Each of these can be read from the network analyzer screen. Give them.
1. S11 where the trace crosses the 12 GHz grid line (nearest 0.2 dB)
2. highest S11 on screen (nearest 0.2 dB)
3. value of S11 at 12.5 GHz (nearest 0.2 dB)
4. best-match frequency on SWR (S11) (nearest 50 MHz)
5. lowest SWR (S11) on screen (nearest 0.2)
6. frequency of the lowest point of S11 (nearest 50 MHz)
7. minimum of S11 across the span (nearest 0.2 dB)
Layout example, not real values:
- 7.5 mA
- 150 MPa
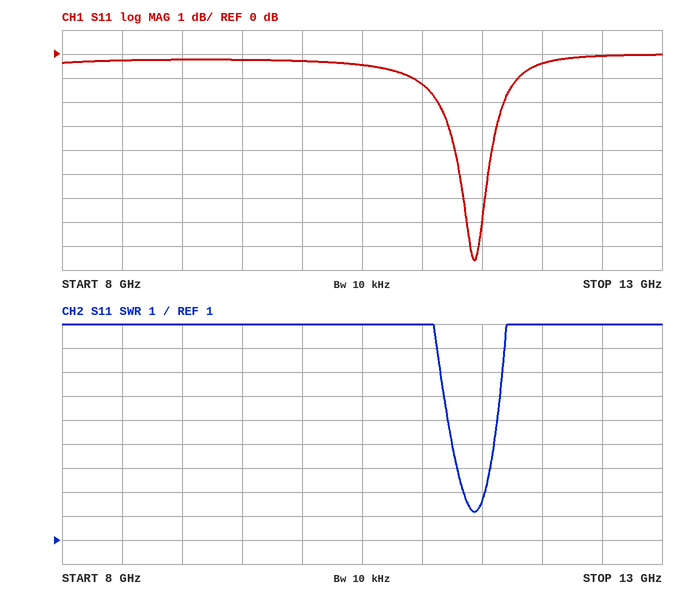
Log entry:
- -0.4 dB
- 0.0 dB
- 0.0 dB
- 11.45 GHz
- 2.2
- 11.45 GHz
- -8.6 dB
